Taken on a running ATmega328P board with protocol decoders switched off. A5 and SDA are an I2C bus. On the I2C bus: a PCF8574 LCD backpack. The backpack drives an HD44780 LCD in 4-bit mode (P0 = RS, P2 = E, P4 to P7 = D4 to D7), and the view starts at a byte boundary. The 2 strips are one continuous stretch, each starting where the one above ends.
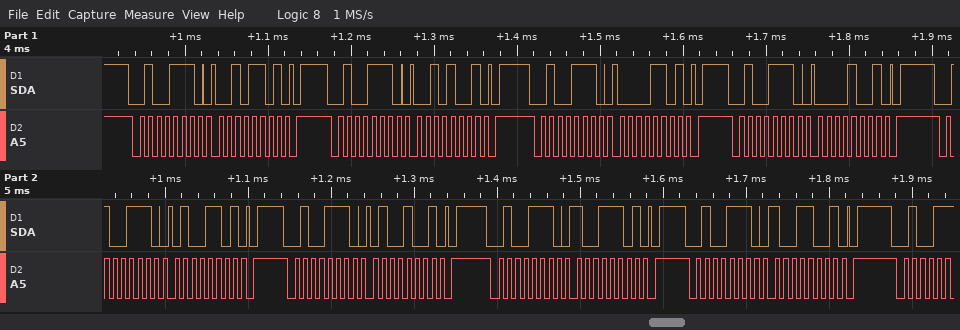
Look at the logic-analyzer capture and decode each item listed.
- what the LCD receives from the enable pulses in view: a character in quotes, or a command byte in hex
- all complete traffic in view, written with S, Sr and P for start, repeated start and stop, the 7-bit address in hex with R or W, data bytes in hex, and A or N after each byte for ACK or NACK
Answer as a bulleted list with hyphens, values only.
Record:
- ' ' 'I'
- S 27W A 2D A P S 27W A 29 A P S 27W A 0D A P S 27W A 09 A P S 27W A 4D A P S 27W A 49 A P S 27W A 9D A P S 27W A 99 A P
